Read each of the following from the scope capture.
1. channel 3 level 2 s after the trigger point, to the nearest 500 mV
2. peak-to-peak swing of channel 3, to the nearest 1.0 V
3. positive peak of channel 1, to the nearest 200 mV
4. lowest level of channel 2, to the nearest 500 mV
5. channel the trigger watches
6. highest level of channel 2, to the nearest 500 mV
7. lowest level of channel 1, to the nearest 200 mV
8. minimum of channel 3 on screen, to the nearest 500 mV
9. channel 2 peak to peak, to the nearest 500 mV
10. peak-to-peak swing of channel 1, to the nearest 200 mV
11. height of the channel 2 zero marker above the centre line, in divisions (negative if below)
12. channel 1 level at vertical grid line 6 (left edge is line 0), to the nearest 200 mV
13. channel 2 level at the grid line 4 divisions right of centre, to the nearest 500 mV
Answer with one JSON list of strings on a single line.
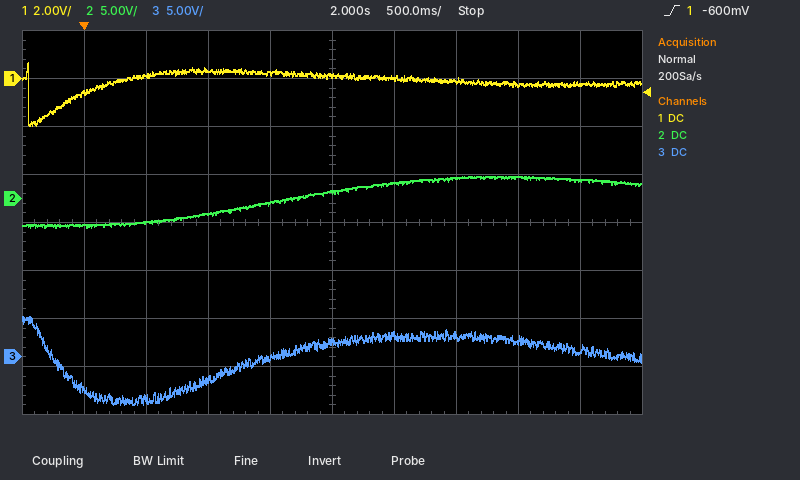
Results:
["1.5 V", "9.0 V", "600 mV", "-3.0 V", "channel 1", "2.5 V", "-2.0 V", "-5.0 V", "5.5 V", "2.6 V", "+0.5 div", "0.0 V", "2.0 V"]
